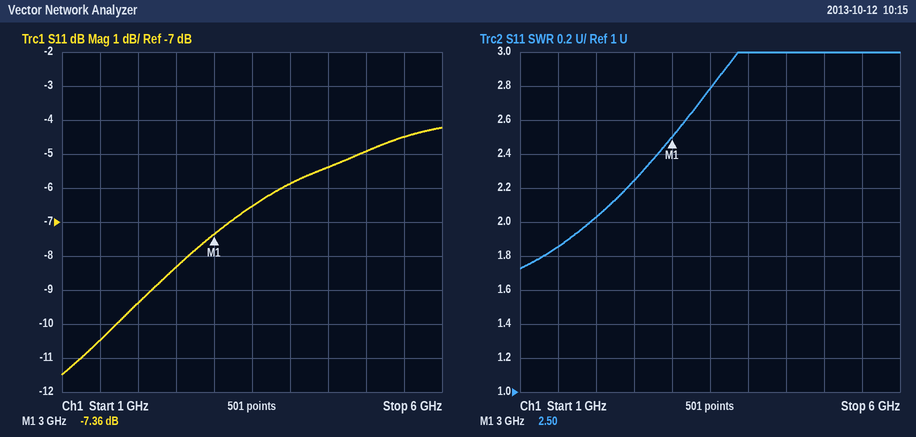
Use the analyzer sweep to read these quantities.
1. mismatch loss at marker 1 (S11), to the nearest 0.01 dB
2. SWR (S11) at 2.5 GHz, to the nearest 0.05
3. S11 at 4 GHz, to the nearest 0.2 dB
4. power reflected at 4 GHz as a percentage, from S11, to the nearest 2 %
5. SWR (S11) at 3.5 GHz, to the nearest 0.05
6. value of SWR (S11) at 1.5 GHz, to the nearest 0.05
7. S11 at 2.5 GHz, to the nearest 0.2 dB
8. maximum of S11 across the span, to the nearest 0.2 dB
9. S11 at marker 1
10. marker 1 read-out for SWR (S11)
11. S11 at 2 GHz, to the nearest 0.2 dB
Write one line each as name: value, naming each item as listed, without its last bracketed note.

mismatch loss at marker 1 (S11), to the nearest 0.01 dB: 0.88 dB
SWR (S11) at 2.5 GHz, to the nearest 0.05: 2.25
S11 at 4 GHz, to the nearest 0.2 dB: -5.8 dB
power reflected at 4 GHz as a percentage, from S11, to the nearest 2 %: 26 %
SWR (S11) at 3.5 GHz, to the nearest 0.05: 2.80
value of SWR (S11) at 1.5 GHz, to the nearest 0.05: 1.85
S11 at 2.5 GHz, to the nearest 0.2 dB: -8.4 dB
maximum of S11 across the span, to the nearest 0.2 dB: -4.2 dB
S11 at marker 1: -7.36 dB
marker 1 read-out for SWR: 2.50
S11 at 2 GHz, to the nearest 0.2 dB: -9.4 dB
